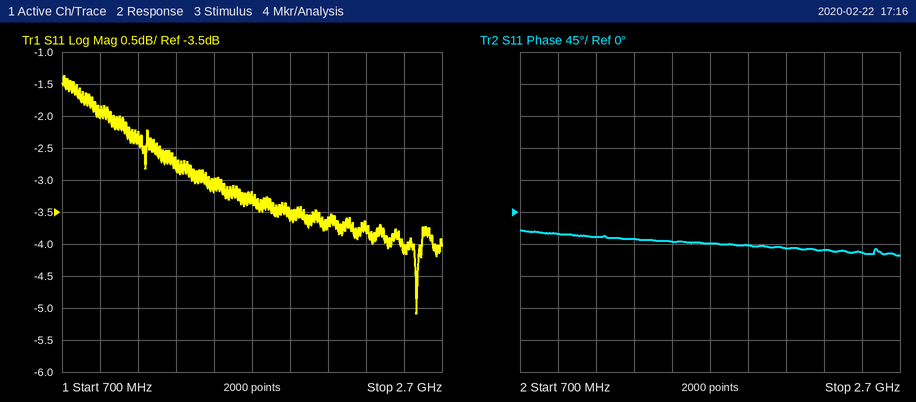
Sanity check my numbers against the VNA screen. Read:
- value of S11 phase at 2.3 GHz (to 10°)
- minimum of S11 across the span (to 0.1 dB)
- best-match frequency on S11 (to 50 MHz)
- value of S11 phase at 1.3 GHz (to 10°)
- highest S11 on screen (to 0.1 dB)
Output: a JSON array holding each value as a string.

["-50°", "-5.1 dB", "2.55 GHz", "-40°", "-1.4 dB"]
